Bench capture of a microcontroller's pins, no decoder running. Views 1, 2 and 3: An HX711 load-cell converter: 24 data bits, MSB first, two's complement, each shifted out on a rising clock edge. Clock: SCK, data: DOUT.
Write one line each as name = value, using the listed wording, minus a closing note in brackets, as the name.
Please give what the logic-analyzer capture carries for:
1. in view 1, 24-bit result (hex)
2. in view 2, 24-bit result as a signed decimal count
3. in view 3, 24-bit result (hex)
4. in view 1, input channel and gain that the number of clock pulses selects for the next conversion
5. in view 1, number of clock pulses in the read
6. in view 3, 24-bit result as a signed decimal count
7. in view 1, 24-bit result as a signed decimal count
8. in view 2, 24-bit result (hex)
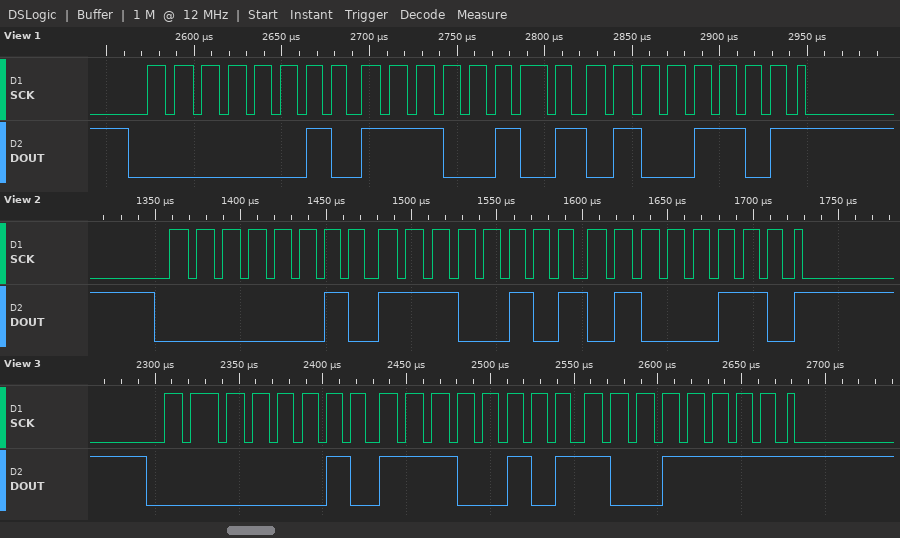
in view 1, 24-bit result = 0x02E54D
in view 2, 24-bit result as a signed decimal count = 189766
in view 3, 24-bit result = 0x02E59F
in view 1, input channel and gain that the number of clock pulses selects for the next conversion = channel A, gain 128
in view 1, number of clock pulses in the read = 25
in view 3, 24-bit result as a signed decimal count = 189855
in view 1, 24-bit result as a signed decimal count = 189773
in view 2, 24-bit result = 0x02E546
